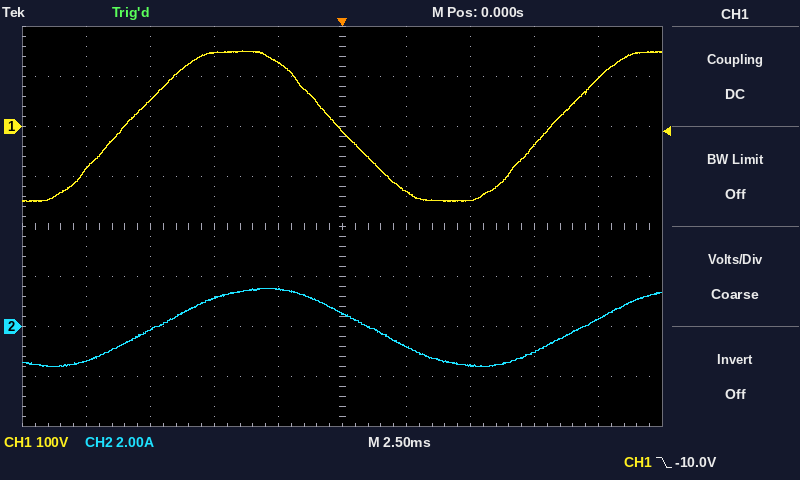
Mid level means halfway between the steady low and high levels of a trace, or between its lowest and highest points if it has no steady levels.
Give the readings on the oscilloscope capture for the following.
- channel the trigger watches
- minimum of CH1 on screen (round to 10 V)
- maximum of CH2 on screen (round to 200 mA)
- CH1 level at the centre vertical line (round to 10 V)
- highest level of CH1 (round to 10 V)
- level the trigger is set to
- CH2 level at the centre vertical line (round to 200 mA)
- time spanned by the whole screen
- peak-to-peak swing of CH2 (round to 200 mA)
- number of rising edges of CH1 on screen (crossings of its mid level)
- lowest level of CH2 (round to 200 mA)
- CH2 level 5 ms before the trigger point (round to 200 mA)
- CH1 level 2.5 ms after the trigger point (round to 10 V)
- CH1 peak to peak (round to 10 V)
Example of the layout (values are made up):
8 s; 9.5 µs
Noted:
CH1; -150 V; 1.6 A; -10 V; 150 V; -10.0 V; 600 mA; 25 ms; 3.2 A; 2; -1.6 A; 1.2 A; -130 V; 300 V
